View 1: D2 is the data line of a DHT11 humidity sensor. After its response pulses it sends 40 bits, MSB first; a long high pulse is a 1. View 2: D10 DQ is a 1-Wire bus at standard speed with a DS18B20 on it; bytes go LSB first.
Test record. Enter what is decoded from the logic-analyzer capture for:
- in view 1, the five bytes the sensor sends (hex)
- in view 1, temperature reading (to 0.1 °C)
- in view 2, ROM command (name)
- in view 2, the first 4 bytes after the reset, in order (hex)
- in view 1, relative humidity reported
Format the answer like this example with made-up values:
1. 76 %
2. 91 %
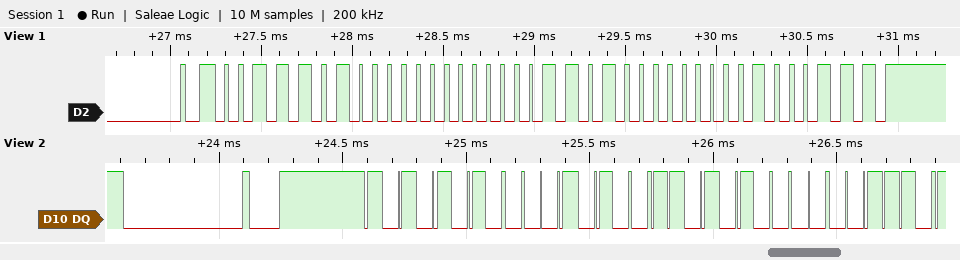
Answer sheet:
1. 3A 00 0D 00 47
2. 13.0 °C
3. Match ROM
4. 55 28 2B 70
5. 58 %
